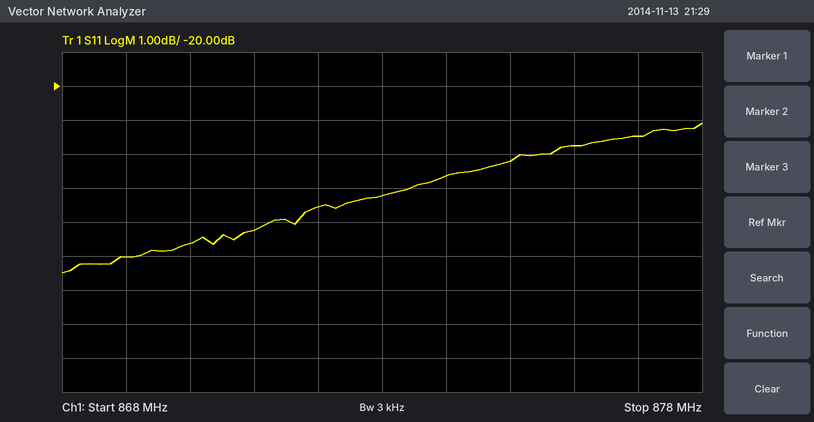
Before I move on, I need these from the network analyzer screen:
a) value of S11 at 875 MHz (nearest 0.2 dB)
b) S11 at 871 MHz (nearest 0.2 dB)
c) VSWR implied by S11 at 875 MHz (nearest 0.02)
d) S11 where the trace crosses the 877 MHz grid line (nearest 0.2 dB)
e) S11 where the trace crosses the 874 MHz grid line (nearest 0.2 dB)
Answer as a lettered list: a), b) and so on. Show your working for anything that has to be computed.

a) -22.2 dB
b) -24.2 dB
c) |Γ| = 10^(-22.2/20) = 0.0776; VSWR = (1 + 0.0776)/(1 − 0.0776) ≈ 1.17, so 1.16 to the nearest 0.02
d) -21.4 dB
e) -22.6 dB
